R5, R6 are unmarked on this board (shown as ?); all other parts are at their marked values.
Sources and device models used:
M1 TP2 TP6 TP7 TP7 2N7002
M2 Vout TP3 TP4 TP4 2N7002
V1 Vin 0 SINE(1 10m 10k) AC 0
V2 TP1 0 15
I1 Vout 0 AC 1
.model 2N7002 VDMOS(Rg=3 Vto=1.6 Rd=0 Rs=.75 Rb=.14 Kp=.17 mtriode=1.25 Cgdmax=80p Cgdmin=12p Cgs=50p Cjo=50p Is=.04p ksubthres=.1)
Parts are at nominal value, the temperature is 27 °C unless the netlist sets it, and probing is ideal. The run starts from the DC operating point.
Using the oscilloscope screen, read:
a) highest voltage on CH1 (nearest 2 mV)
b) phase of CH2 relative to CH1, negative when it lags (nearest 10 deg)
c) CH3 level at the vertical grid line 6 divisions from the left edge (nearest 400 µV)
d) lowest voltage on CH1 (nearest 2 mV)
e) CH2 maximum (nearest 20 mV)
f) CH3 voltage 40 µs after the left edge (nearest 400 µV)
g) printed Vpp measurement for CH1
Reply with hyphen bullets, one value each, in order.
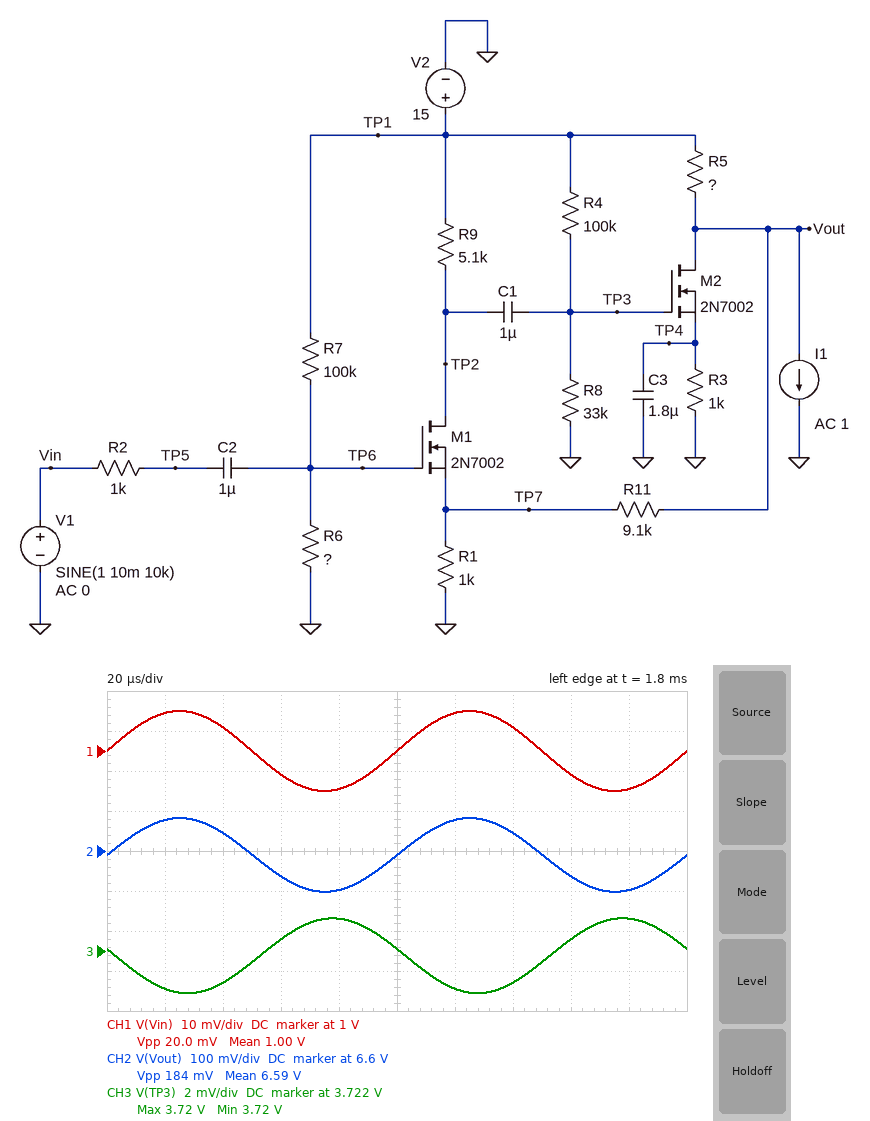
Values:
- 1.010 V
- 0 deg
- 3.7200 V
- 990 mV
- 6.68 V
- 3.7204 V
- 20.0 mV
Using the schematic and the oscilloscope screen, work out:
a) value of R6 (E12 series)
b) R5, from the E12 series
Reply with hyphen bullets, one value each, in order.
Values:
- 27 kΩ
- 3.3 kΩ
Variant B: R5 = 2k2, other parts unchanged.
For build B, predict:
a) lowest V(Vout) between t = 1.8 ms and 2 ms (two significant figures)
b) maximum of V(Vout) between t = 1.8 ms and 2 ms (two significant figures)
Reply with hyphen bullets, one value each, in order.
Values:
- 8.8 V
- 8.9 V
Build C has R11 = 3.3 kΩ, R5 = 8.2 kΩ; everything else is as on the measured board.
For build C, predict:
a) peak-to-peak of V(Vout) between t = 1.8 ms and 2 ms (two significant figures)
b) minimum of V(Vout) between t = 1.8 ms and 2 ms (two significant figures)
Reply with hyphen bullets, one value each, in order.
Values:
- 2.7 mV
- 1.6 V
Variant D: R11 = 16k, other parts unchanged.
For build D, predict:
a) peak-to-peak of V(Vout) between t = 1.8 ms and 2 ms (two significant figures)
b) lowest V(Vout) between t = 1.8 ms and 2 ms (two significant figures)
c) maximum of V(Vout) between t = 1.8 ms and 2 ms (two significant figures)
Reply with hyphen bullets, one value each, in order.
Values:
- 300 mV
- 7.1 V
- 7.4 V
